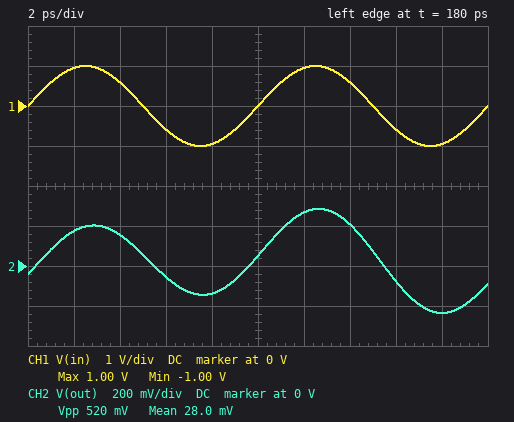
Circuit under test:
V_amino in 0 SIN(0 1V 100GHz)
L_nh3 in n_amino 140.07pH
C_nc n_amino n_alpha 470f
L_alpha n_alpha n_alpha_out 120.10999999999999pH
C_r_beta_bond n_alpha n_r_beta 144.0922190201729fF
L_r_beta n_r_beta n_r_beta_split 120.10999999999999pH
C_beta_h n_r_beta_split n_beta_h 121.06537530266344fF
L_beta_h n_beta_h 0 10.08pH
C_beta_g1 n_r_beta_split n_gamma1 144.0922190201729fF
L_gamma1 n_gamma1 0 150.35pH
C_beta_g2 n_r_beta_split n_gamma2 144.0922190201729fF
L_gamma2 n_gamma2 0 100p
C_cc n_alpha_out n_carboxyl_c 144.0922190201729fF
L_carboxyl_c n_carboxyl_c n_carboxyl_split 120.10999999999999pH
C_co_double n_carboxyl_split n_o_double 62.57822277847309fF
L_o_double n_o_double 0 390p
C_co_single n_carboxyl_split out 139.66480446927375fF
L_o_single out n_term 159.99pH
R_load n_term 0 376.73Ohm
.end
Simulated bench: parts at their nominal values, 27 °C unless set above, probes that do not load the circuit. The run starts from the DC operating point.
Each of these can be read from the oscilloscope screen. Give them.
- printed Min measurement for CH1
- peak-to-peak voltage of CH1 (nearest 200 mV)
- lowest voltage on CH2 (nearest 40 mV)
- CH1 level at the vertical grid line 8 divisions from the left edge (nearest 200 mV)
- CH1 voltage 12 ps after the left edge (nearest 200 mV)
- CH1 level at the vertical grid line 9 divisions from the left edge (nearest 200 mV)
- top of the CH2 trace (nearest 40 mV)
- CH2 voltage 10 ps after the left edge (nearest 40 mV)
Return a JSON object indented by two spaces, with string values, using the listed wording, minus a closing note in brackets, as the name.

{
  "printed Min measurement for CH1": "-1.00 V",
  "peak-to-peak voltage of CH1": "2.0 V",
  "lowest voltage on CH2": "-240 mV",
  "CH1 level at the vertical grid line 8 divisions from the left edge": "-600 mV",
  "CH1 voltage 12 ps after the left edge": "1.0 V",
  "CH1 level at the vertical grid line 9 divisions from the left edge": "-1.0 V",
  "top of the CH2 trace": "280 mV",
  "CH2 voltage 10 ps after the left edge": "40 mV"
}
